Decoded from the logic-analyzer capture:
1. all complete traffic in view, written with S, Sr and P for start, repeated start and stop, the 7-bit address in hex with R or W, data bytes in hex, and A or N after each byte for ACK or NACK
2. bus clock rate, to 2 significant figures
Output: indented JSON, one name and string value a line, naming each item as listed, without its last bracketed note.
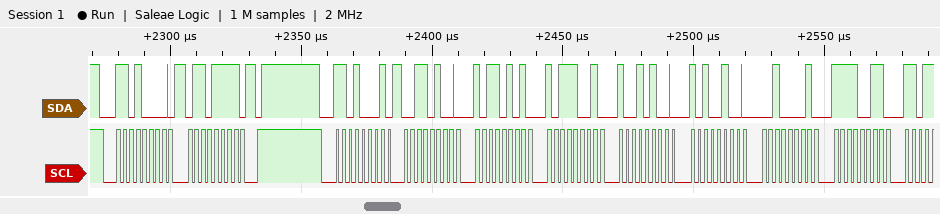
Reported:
{
  "all complete traffic in view, written with S, Sr and P for start, repeated start and stop, the 7-bit address in hex with R or W, data bytes in hex, and A or N after each byte for ACK or NACK": "S 68W A 6F A P S 68R A 34 A B5 A B9 A 94 A A4 A 21 A F3 A",
  "bus clock rate, to 2 significant figures": "400 kHz"
}
